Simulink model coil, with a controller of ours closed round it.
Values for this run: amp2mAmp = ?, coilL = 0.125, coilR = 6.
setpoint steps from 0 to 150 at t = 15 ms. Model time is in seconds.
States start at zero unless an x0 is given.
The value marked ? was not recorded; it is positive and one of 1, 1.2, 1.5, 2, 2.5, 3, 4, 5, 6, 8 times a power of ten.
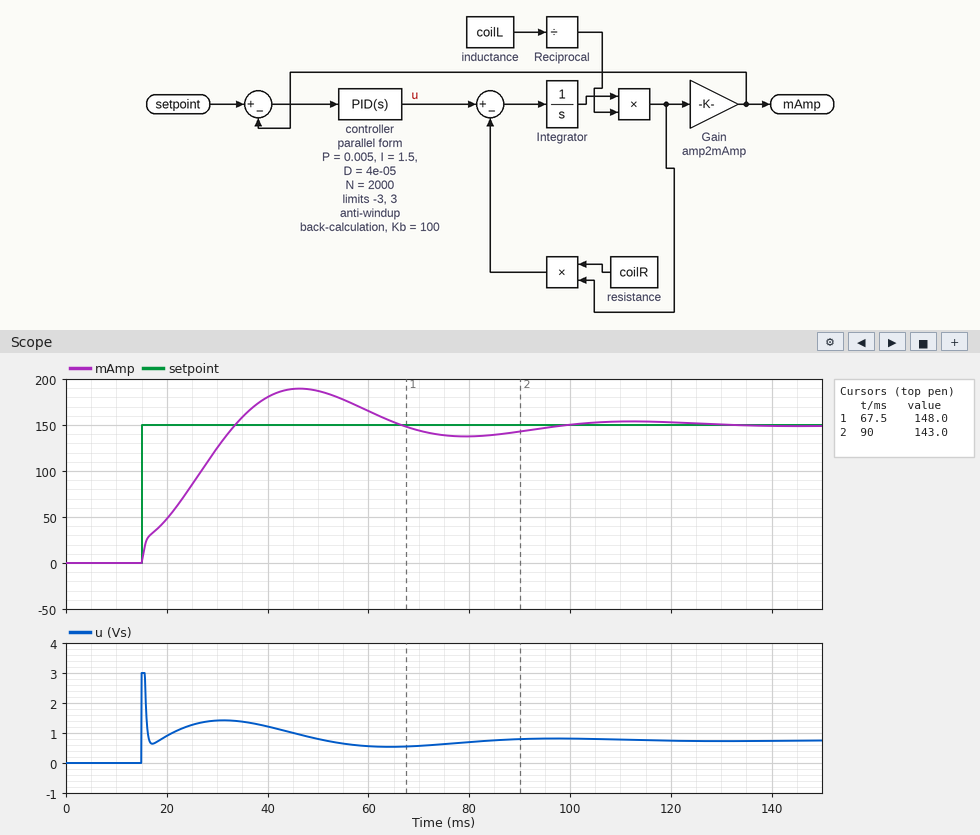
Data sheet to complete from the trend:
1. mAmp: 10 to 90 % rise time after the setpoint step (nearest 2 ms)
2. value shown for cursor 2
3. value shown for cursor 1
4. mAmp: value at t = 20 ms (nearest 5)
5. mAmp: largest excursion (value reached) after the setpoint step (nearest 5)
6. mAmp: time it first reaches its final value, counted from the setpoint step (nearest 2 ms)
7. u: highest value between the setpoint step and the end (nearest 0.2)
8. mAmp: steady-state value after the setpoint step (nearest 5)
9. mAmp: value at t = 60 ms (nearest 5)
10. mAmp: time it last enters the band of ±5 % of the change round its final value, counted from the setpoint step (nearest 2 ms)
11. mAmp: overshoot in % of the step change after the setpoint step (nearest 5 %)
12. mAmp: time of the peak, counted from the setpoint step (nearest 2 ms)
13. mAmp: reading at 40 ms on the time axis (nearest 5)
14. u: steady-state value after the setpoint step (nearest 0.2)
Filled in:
16 ms
143.0
148.0
50
190
18 ms
3.0
150
165
74 ms
25 %
32 ms
180
0.8
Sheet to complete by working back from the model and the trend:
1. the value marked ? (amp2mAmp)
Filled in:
1200
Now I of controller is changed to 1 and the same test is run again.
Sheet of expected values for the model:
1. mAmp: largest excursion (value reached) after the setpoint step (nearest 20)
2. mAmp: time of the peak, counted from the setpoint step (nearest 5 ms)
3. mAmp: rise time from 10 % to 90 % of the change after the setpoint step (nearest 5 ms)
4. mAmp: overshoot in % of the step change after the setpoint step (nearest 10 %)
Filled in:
180
40 ms
20 ms
20 %
